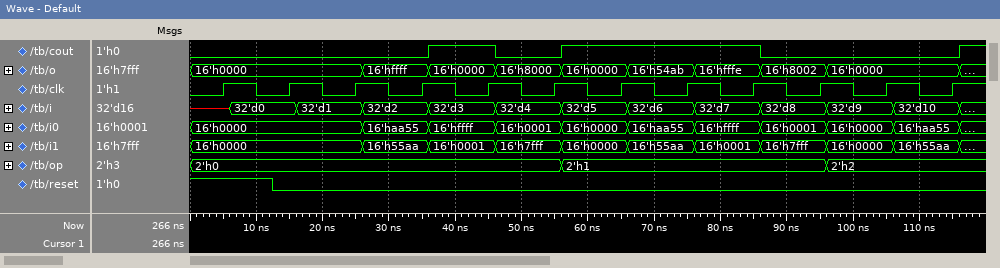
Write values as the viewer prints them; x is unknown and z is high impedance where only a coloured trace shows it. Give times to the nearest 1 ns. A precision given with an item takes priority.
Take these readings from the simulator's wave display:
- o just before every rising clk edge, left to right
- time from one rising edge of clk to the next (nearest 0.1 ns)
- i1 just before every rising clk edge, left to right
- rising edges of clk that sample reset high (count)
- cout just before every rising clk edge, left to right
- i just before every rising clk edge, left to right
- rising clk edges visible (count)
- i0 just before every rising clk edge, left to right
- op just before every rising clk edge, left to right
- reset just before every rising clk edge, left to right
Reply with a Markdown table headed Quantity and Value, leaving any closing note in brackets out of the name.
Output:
| Quantity | Value |
|---|---|
| o just before every rising clk edge, left to right | 16'h0000, 16'h0000, 16'h0000, 16'hffff, 16'h0000, 16'h8000, 16'h0000, 16'h54ab, 16'hfffe, 16'h8002, 16'h0000, 16'h0000 |
| time from one rising edge of clk to the next | 10 ns |
| i1 just before every rising clk edge, left to right | 16'h0000, 16'h0000, 16'h0000, 16'h55aa, 16'h0001, 16'h7fff, 16'h0000, 16'h55aa, 16'h0001, 16'h7fff, 16'h0000, 16'h55aa |
| rising edges of clk that sample reset high | 1 |
| cout just before every rising clk edge, left to right | 0 0 0 0 1 0 1 1 1 0 0 0 |
| i just before every rising clk edge, left to right | x, 32'd0, 32'd1, 32'd2, 32'd3, 32'd4, 32'd5, 32'd6, 32'd7, 32'd8, 32'd9, 32'd10 |
| rising clk edges visible | 12 |
| i0 just before every rising clk edge, left to right | 16'h0000, 16'h0000, 16'h0000, 16'haa55, 16'hffff, 16'h0001, 16'h0000, 16'haa55, 16'hffff, 16'h0001, 16'h0000, 16'haa55 |
| op just before every rising clk edge, left to right | 2'h0, 2'h0, 2'h0, 2'h0, 2'h0, 2'h0, 2'h1, 2'h1, 2'h1, 2'h1, 2'h2, 2'h2 |
| reset just before every rising clk edge, left to right | 1 0 0 0 0 0 0 0 0 0 0 0 |
